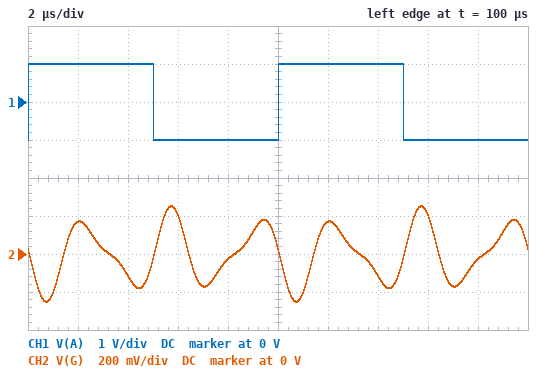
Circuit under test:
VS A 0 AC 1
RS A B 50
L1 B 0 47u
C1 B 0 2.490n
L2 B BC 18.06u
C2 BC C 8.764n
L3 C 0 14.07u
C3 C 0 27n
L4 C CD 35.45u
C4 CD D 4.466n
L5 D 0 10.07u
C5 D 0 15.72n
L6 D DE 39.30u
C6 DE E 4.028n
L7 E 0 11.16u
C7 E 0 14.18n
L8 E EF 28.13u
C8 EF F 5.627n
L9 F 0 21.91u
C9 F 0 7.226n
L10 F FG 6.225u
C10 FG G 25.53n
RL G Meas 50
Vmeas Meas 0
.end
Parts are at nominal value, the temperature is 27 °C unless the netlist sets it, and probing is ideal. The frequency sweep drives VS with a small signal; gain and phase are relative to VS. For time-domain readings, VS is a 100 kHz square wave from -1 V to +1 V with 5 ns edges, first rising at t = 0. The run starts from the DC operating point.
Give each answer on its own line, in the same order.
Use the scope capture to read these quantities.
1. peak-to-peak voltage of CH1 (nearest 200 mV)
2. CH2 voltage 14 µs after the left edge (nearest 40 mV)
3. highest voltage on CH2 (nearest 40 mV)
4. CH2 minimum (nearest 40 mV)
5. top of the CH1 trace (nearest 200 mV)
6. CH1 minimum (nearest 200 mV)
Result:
2.0 V
-120 mV
240 mV
-240 mV
1.0 V
-1.0 V
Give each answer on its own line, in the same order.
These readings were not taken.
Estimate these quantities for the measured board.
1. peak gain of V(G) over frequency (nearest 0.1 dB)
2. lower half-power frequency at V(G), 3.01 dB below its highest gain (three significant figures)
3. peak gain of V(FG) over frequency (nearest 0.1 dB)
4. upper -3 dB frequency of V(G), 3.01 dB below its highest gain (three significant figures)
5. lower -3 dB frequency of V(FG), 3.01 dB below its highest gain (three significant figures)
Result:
-7.8 dB
256 kHz
-7.1 dB
523 kHz
255 kHz
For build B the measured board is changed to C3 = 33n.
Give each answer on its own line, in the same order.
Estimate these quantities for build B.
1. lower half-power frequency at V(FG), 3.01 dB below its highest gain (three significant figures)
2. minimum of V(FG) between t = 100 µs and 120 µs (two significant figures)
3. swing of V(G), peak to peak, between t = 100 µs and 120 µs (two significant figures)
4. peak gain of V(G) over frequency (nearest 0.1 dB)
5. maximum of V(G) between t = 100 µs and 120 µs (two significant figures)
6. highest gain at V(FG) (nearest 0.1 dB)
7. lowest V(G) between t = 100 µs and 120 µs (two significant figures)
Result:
256 kHz
-220 mV
420 mV
-9.0 dB
210 mV
-8.2 dB
-210 mV
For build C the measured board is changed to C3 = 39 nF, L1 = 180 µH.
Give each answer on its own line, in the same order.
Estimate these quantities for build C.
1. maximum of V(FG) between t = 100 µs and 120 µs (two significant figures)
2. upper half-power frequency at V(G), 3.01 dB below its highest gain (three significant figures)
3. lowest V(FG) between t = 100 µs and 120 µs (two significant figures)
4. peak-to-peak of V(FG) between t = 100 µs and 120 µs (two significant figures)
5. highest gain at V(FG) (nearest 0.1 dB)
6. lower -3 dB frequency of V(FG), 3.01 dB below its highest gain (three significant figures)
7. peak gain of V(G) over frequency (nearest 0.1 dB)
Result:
160 mV
556 kHz
-160 mV
320 mV
-10.9 dB
257 kHz
-11.7 dB
